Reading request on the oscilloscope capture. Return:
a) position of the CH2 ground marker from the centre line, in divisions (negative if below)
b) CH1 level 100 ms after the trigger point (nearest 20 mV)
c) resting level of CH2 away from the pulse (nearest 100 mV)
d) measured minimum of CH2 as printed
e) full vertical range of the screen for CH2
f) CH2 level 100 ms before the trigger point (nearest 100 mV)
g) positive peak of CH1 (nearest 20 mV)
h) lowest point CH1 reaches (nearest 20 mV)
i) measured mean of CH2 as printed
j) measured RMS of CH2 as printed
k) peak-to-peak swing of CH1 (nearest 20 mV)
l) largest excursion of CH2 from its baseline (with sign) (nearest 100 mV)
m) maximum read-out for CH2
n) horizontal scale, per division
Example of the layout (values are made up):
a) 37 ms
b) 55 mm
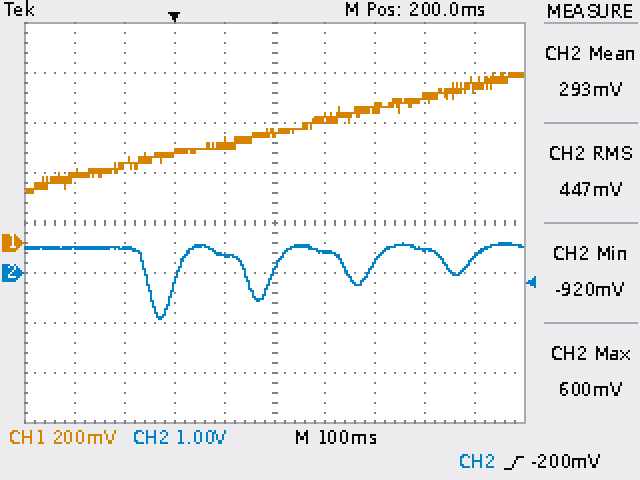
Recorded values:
a) -1.0 div
b) 400 mV
c) 500 mV
d) -920 mV
e) 8 V
f) 500 mV
g) 680 mV
h) 200 mV
i) 293 mV
j) 447 mV
k) 480 mV
l) -1.4 V
m) 600 mV
n) 100 ms
